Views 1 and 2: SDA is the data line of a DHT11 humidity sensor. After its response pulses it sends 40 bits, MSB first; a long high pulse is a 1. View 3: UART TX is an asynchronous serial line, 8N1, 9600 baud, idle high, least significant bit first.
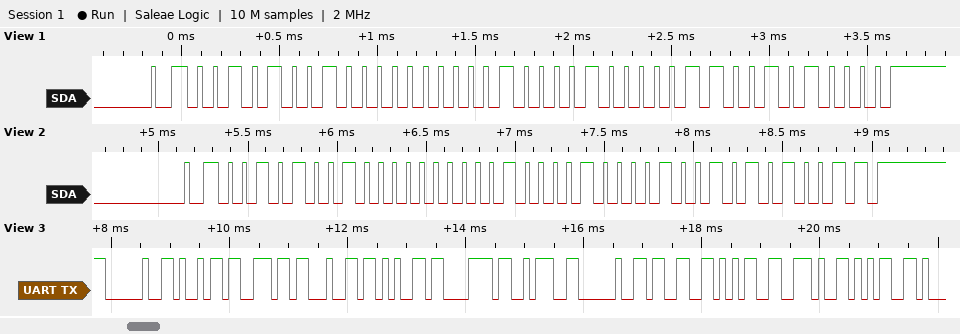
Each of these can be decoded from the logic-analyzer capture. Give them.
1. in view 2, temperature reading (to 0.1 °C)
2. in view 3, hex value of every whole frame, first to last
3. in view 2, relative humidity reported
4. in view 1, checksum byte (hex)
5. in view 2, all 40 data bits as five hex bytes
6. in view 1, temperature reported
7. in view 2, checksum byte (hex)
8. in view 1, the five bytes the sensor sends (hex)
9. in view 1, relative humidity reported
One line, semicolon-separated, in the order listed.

33.9 °C; 20 69 6E 64 65 78 3A 20 33 35 2E 35; 41 %; 0x50; 29 00 21 09 53; 33.6 °C; 0x53; 29 00 21 06 50; 41 %
